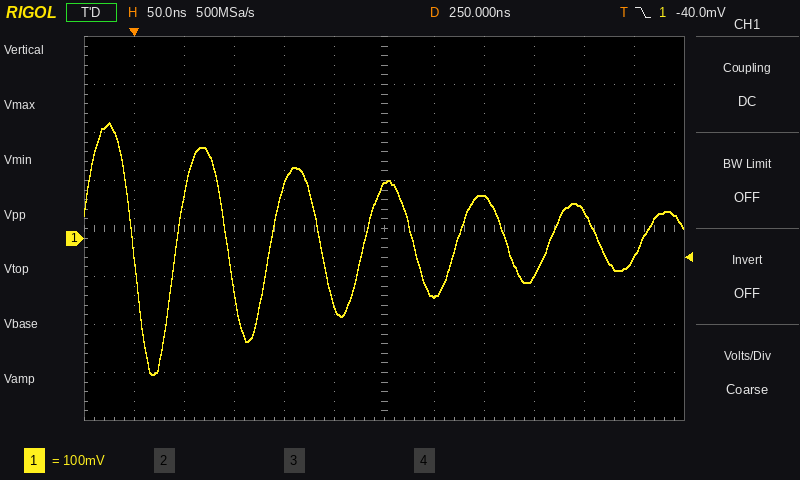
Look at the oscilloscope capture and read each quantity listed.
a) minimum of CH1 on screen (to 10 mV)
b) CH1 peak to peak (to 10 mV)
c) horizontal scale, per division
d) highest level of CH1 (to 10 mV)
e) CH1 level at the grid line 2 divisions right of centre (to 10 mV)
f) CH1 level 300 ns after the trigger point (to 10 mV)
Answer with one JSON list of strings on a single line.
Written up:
["-280 mV", "520 mV", "50 ns", "240 mV", "90 mV", "-120 mV"]
